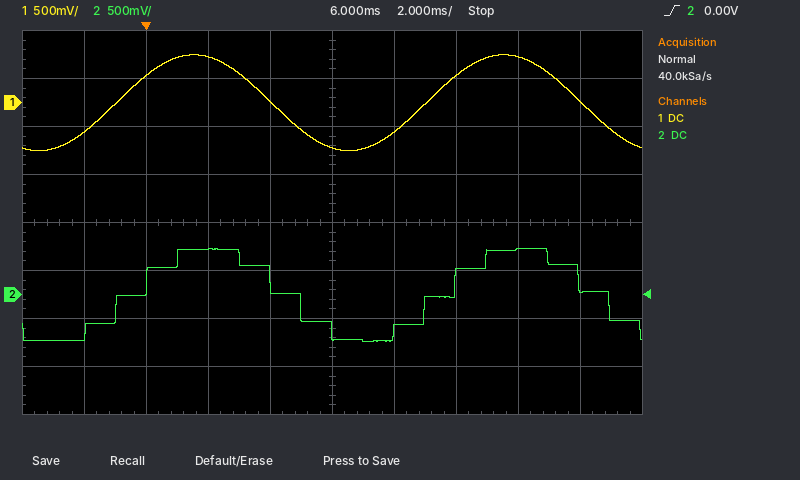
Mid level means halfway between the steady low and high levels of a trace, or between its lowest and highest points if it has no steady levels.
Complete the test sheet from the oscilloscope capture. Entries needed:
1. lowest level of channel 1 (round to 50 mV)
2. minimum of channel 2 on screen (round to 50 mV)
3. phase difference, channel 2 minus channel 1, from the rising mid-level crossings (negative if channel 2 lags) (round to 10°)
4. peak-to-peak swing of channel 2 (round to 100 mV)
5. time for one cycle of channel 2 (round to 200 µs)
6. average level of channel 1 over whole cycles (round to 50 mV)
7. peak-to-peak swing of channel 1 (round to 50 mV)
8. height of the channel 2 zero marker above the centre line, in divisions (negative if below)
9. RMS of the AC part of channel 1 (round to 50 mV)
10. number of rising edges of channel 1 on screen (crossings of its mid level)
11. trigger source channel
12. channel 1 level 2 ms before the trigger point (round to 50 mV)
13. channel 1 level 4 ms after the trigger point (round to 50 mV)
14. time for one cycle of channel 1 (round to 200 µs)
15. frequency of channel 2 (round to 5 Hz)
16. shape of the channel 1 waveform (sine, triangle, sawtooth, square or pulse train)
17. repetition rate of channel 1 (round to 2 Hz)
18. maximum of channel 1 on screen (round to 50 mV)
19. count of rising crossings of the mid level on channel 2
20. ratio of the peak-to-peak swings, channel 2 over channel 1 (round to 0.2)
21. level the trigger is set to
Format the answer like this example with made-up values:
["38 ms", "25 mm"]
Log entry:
["-500 mV", "-500 mV", "-30°", "1.00 V", "10.0 ms", "0 mV", "1.00 V", "-1.5 div", "350 mV", "2", "channel 2", "-300 mV", "0 mV", "10.0 ms", "100 Hz", "sine", "100 Hz", "500 mV", "2", "1.0", "0.00 V"]
